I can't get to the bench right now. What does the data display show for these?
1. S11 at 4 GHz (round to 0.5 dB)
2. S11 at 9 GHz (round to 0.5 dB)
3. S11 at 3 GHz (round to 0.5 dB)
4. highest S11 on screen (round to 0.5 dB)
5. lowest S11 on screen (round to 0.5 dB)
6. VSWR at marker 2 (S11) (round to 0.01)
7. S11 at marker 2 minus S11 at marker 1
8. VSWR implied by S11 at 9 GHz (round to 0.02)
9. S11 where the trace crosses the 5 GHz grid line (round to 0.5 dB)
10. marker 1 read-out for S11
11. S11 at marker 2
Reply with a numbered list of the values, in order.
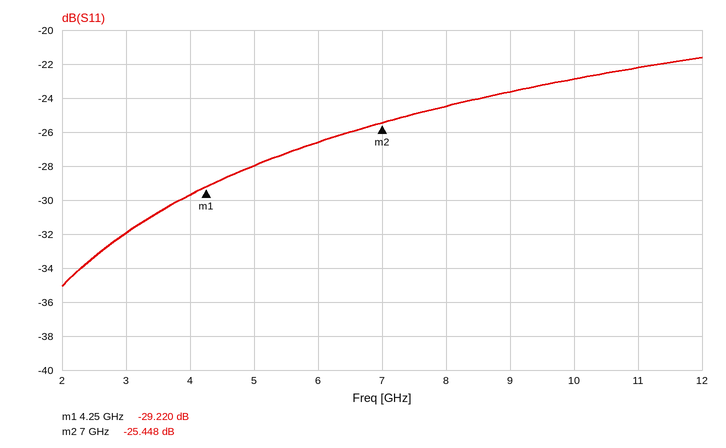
1. -29.5 dB
2. -23.5 dB
3. -32.0 dB
4. -21.5 dB
5. -35.0 dB
6. 1.11
7. 3.772 dB
8. 1.14
9. -28.0 dB
10. -29.220 dB
11. -25.448 dB
